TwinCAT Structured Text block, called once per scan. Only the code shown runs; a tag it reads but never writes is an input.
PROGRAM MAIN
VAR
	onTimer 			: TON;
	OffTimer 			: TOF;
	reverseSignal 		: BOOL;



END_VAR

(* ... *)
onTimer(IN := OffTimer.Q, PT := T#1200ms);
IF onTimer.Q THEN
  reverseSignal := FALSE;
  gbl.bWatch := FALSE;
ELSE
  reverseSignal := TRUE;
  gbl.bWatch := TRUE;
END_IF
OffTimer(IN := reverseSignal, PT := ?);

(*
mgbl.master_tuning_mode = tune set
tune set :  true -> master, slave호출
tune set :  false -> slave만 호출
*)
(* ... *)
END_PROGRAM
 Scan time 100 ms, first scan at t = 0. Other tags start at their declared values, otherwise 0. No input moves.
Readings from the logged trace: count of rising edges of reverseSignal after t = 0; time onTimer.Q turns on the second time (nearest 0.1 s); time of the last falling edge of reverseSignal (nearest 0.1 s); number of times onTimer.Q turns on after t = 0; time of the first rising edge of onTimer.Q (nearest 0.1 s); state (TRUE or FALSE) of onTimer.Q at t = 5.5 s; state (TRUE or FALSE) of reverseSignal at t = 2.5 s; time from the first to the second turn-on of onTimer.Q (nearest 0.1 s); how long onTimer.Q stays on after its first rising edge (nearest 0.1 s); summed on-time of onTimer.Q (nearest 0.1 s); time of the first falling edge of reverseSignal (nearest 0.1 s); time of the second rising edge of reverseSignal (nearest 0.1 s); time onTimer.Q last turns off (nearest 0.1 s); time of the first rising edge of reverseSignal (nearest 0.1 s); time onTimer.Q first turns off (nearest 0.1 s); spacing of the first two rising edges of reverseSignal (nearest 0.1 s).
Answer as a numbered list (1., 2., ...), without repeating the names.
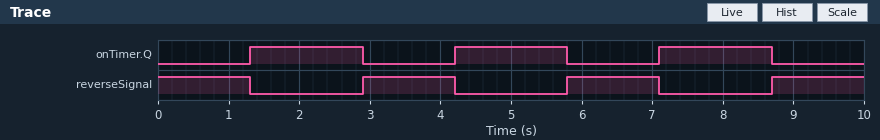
1. 3
2. 4.2 s
3. 7.1 s
4. 3
5. 1.3 s
6. TRUE
7. FALSE
8. 2.9 s
9. 1.6 s
10. 4.8 s
11. 1.3 s
12. 5.8 s
13. 8.7 s
14. 2.9 s
15. 2.9 s
16. 2.9 s
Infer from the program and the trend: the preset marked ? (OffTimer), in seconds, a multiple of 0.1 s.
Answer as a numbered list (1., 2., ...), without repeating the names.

1. 1.5 s
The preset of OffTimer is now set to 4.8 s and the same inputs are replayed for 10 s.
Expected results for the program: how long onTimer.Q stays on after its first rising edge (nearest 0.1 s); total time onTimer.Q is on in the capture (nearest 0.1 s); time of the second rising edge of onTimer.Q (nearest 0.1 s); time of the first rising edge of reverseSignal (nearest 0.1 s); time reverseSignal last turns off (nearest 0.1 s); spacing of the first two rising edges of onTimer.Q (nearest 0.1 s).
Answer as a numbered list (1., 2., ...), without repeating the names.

1. 4.9 s
2. 7.4 s
3. 7.5 s
4. 6.2 s
5. 7.5 s
6. 6.2 s
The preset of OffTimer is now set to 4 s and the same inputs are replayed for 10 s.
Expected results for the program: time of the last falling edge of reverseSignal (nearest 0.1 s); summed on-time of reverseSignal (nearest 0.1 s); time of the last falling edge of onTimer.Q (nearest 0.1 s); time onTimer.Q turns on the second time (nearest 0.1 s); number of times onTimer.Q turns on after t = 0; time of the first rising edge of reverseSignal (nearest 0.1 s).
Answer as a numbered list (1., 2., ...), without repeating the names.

1. 6.7 s
2. 2.6 s
3. 5.4 s
4. 6.7 s
5. 2
6. 5.4 s
